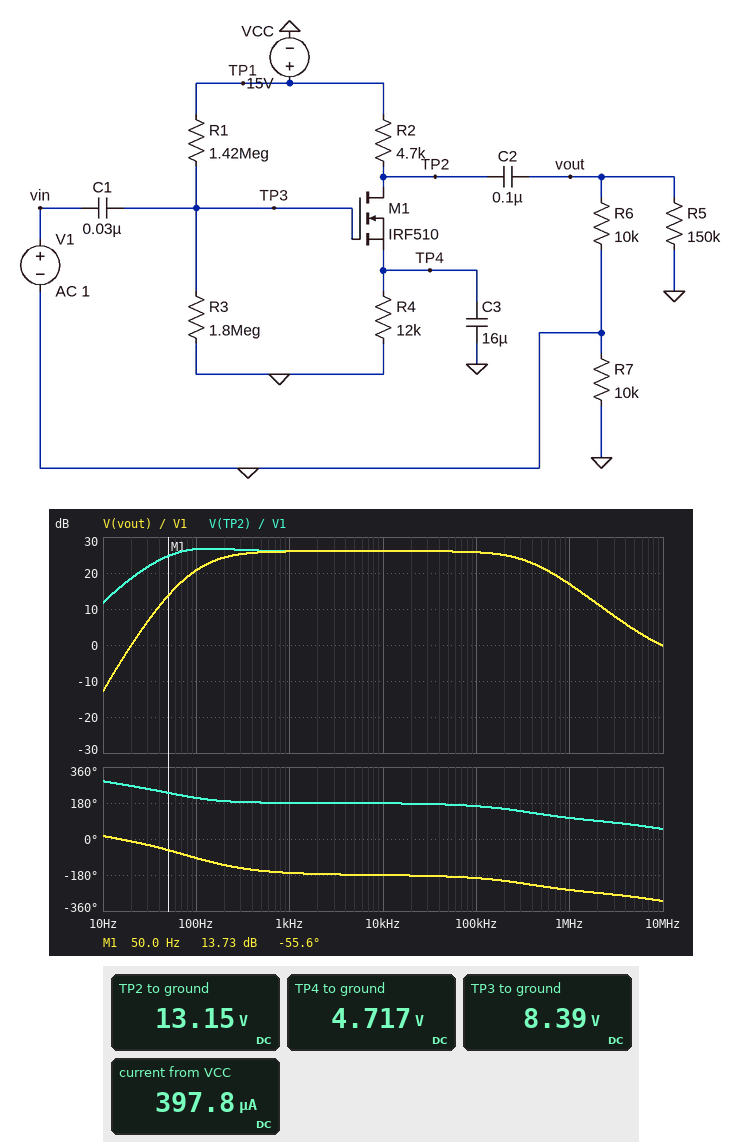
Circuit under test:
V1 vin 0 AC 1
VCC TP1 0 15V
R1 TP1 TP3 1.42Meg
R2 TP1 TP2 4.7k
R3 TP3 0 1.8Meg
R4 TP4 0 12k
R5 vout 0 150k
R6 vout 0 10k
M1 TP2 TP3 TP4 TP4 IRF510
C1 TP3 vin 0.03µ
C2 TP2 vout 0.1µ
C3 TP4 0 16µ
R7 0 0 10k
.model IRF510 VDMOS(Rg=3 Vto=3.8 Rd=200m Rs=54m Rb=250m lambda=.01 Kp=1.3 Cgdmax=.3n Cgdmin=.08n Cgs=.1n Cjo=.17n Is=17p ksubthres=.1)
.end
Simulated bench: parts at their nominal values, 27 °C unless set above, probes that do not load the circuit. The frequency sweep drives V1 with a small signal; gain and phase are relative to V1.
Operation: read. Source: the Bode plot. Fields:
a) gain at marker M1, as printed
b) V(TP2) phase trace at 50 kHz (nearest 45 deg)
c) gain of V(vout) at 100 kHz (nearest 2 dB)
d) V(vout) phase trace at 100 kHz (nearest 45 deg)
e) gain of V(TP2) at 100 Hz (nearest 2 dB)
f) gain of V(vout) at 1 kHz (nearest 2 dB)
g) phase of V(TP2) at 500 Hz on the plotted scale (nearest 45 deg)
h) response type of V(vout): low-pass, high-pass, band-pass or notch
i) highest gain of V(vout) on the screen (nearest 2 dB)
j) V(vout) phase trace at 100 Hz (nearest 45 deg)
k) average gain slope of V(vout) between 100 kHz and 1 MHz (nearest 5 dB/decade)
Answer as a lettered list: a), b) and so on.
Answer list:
a) 13.73 dB
b) 180 deg
c) 26 dB
d) -180 deg
e) 26 dB
f) 26 dB
g) 180 deg
h) band-pass
i) 26 dB
j) -90 deg
k) -10 dB/decade
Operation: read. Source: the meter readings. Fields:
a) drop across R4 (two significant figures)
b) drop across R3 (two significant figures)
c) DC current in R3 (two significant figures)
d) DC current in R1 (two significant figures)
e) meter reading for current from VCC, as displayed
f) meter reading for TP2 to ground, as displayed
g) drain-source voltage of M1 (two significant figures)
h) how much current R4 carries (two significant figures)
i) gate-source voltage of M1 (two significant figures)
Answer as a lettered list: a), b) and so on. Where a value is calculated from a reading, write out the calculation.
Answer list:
a) 4.717 V = 4.7 V
b) 8.39 V = 8.4 V
c) (8.39 V) / 1.8 MΩ = 4.7 µA
d) (15 V - 8.39 V) / 1.42 MΩ = 4.7 µA
e) 397.8 µA
f) 13.15 V
g) 13.15 V - 4.717 V = 8.4 V
h) (4.717 V) / 12 kΩ = 390 µA
i) 8.39 V - 4.717 V = 3.7 V
